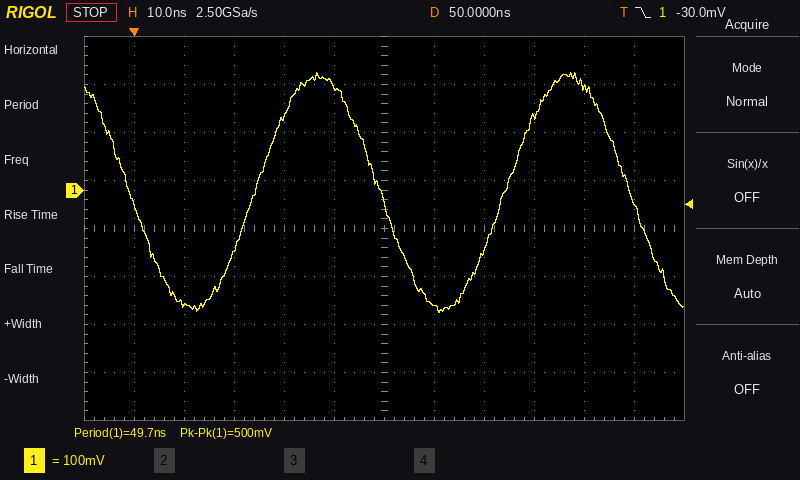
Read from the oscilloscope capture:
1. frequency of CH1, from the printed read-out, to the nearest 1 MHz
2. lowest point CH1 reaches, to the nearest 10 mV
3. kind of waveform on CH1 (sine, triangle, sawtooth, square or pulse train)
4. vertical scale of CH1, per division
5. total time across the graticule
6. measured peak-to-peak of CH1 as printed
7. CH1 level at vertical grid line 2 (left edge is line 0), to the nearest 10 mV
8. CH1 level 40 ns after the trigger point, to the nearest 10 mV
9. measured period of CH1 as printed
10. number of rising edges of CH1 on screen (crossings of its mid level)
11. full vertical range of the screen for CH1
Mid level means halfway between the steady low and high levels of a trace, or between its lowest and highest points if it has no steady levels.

20 MHz
-260 mV
sine
100 mV
120 ns
500 mV
-240 mV
220 mV
49.7 ns
2
800 mV
